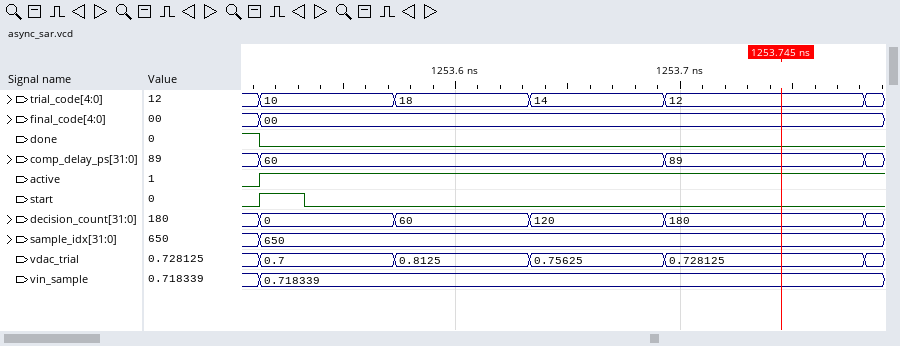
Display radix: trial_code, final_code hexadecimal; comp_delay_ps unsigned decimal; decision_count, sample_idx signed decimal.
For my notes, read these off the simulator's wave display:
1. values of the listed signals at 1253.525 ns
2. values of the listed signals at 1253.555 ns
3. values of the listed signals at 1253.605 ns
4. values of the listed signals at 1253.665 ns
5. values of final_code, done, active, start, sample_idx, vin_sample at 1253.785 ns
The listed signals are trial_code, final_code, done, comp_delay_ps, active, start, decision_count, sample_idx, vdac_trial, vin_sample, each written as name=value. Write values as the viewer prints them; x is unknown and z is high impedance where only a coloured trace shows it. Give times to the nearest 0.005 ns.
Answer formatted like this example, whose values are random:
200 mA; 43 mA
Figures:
trial_code=10, final_code=00, done=0, comp_delay_ps=60, active=1, start=1, decision_count=0, sample_idx=650, vdac_trial=0.7, vin_sample=0.718339; trial_code=10, final_code=00, done=0, comp_delay_ps=60, active=1, start=0, decision_count=0, sample_idx=650, vdac_trial=0.7, vin_sample=0.718339; trial_code=18, final_code=00, done=0, comp_delay_ps=60, active=1, start=0, decision_count=60, sample_idx=650, vdac_trial=0.8125, vin_sample=0.718339; trial_code=14, final_code=00, done=0, comp_delay_ps=60, active=1, start=0, decision_count=120, sample_idx=650, vdac_trial=0.75625, vin_sample=0.718339; final_code=00, done=0, active=1, start=0, sample_idx=650, vin_sample=0.718339
